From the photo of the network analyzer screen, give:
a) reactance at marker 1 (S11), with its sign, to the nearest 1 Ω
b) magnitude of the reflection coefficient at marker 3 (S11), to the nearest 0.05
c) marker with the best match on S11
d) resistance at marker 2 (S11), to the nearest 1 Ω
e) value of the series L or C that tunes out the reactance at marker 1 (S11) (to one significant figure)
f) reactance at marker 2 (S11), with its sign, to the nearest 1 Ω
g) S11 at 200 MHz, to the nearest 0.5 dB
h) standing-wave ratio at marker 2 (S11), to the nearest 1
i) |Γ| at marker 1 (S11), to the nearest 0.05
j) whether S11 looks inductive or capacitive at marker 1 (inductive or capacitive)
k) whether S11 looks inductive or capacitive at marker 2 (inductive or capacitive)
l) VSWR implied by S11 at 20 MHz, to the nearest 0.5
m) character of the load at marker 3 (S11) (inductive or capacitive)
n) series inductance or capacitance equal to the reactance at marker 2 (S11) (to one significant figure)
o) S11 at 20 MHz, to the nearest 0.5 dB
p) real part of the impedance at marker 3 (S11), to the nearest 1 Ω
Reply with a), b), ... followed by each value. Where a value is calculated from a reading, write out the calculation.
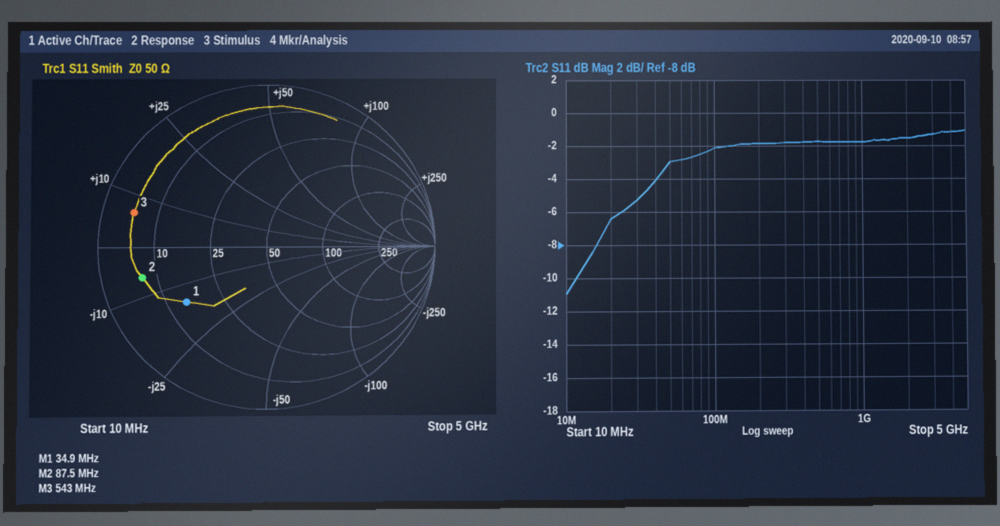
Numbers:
a) -15 Ω
b) 0.80
c) marker 1
d) 7 Ω
e) L = 15 Ω/(2π × 34.9 MHz) ≈ 68.4 nH, so 70 nH to one significant figure
f) -6 Ω
g) -2.0 dB
h) 7
i) 0.60
j) capacitive
k) capacitive
l) |Γ| = 10^(-6.5/20) = 0.4732; VSWR = (1 + 0.4732)/(1 − 0.4732) ≈ 2.80, so 3.0 to the nearest 0.5
m) inductive
n) C = 1/(2π × 87.5 MHz × 6 Ω) ≈ 303 pF, so 300 pF to one significant figure
o) -6.5 dB
p) 5 Ω
